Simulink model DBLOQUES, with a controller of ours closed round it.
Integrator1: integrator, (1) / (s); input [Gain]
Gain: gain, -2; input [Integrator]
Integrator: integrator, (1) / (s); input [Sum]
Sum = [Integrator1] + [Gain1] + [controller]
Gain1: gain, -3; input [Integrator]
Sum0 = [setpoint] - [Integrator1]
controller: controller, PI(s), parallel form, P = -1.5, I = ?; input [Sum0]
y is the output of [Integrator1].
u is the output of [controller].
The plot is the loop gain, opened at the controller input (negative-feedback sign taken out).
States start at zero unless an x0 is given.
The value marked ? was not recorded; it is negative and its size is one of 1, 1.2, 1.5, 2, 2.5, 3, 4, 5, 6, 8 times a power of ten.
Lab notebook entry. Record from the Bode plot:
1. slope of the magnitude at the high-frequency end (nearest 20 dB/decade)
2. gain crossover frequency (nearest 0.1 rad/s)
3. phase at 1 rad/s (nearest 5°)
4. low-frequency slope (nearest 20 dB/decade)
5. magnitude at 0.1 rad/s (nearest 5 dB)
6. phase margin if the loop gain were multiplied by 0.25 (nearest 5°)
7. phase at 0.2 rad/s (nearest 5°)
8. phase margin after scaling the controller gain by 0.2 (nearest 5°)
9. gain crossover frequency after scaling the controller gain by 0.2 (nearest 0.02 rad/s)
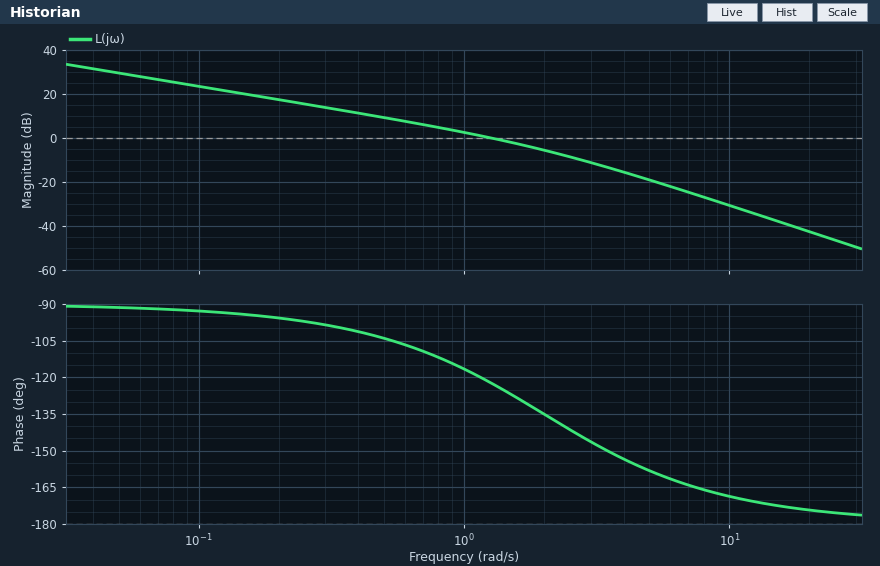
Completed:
-40 dB/decade
1.3 rad/s
-115°
-20 dB/decade
25 dB
80°
-95°
80°
0.30 rad/s
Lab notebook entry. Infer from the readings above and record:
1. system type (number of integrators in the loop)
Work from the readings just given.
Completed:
1
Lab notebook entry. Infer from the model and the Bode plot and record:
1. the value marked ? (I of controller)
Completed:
-1.5
